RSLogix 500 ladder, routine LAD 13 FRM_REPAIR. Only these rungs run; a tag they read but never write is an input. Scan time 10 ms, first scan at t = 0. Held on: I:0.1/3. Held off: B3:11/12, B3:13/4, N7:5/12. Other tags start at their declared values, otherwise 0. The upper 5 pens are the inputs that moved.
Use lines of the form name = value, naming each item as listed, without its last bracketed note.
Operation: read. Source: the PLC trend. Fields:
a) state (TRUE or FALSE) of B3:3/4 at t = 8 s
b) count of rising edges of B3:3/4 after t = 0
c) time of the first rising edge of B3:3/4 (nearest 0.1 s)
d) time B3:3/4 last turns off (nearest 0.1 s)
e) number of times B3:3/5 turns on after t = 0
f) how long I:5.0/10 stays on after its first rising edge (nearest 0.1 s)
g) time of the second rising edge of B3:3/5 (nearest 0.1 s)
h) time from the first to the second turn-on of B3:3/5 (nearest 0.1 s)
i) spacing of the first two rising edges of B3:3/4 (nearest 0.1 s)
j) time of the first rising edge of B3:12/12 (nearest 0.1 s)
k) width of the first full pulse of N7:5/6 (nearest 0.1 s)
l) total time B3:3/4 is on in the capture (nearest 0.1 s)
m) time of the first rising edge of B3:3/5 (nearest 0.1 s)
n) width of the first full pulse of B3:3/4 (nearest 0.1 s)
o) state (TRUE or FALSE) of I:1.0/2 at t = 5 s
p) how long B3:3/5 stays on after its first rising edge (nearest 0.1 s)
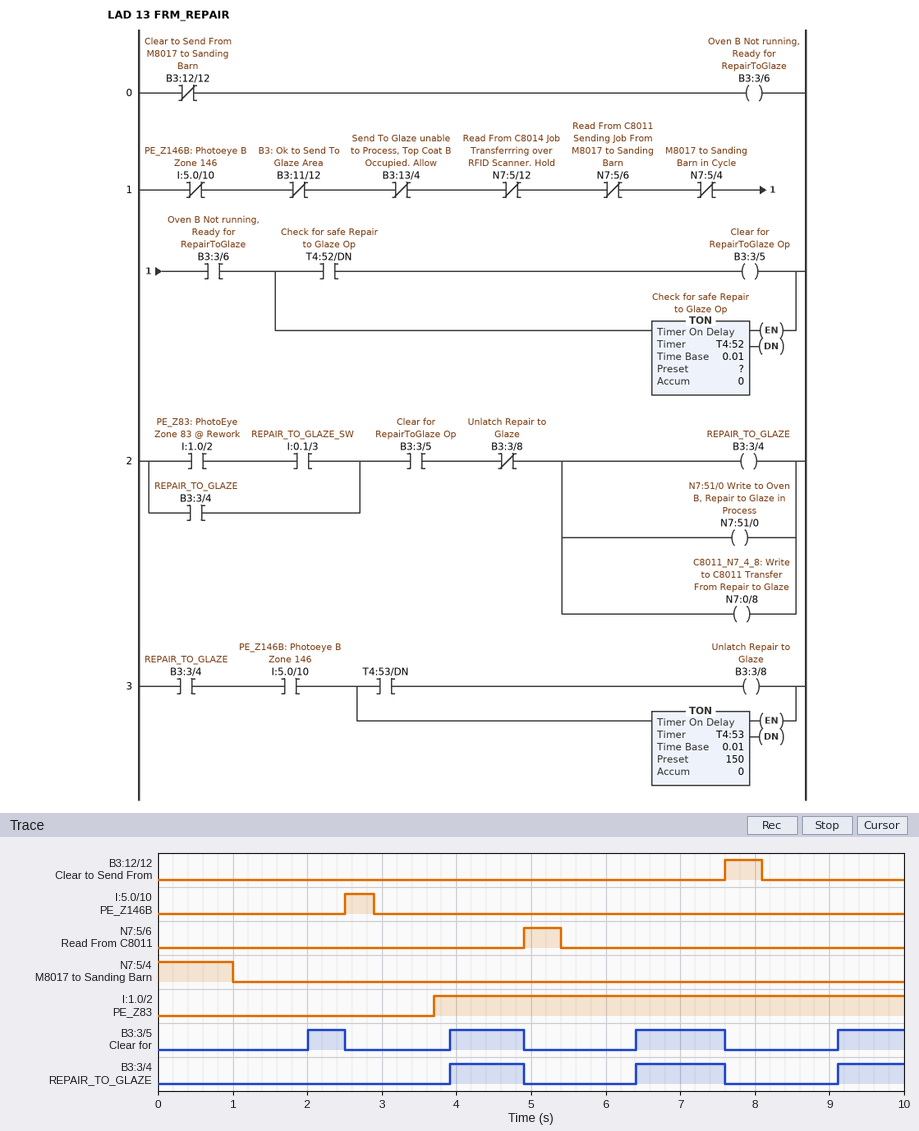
state (TRUE or FALSE) of B3:3/4 at t = 8 s = FALSE
count of rising edges of B3:3/4 after t = 0 = 3
time of the first rising edge of B3:3/4 = 3.9 s
time B3:3/4 last turns off = 7.6 s
number of times B3:3/5 turns on after t = 0 = 4
how long I:5.0/10 stays on after its first rising edge = 0.4 s
time of the second rising edge of B3:3/5 = 3.9 s
time from the first to the second turn-on of B3:3/5 = 1.9 s
spacing of the first two rising edges of B3:3/4 = 2.5 s
time of the first rising edge of B3:12/12 = 7.6 s
width of the first full pulse of N7:5/6 = 0.5 s
total time B3:3/4 is on in the capture = 3.1 s
time of the first rising edge of B3:3/5 = 2.0 s
width of the first full pulse of B3:3/4 = 1.0 s
state (TRUE or FALSE) of I:1.0/2 at t = 5 s = TRUE
how long B3:3/5 stays on after its first rising edge = 0.5 s
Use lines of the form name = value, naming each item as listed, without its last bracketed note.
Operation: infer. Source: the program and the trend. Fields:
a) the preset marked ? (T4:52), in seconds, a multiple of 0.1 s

the preset marked ? (T4:52), in seconds, a multiple of 0.1 s = 1.0 s
